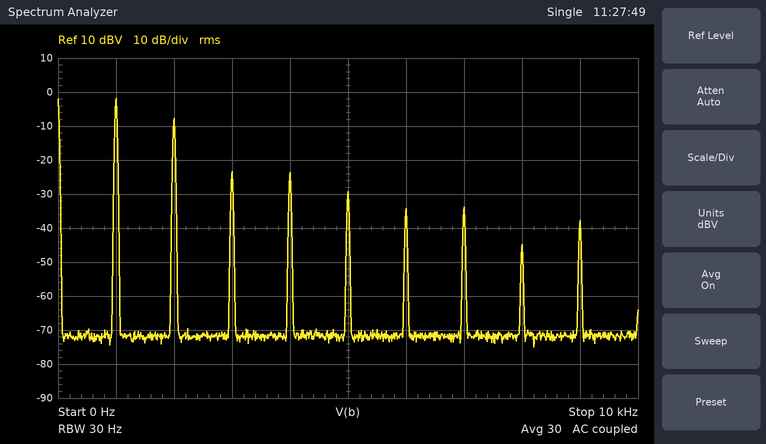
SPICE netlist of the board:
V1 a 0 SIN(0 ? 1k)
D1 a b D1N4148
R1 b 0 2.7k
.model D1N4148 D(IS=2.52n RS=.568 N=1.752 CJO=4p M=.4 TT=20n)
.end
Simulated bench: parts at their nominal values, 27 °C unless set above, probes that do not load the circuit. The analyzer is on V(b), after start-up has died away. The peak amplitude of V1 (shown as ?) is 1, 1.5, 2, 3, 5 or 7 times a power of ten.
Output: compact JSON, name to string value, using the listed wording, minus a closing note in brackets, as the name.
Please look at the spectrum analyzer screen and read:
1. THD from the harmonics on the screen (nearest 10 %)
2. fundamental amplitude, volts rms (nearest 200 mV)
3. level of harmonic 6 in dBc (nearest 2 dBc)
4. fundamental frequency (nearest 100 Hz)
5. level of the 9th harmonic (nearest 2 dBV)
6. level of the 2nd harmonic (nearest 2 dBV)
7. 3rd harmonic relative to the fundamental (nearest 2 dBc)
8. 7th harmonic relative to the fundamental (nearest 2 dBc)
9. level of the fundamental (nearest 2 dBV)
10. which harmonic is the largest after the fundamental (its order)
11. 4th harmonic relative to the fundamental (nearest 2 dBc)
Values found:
{"THD from the harmonics on the screen": "50 %", "fundamental amplitude, volts rms": "800 mV", "level of harmonic 6 in dBc": "-32 dBc", "fundamental frequency": "1.0 kHz", "level of the 9th harmonic": "-38 dBV", "level of the 2nd harmonic": "-8 dBV", "3rd harmonic relative to the fundamental": "-22 dBc", "7th harmonic relative to the fundamental": "-32 dBc", "level of the fundamental": "-2 dBV", "which harmonic is the largest after the fundamental": "2", "4th harmonic relative to the fundamental": "-22 dBc"}
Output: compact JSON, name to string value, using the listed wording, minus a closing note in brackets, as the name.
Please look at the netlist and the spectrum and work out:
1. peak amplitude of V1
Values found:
{"peak amplitude of V1": "3 V"}
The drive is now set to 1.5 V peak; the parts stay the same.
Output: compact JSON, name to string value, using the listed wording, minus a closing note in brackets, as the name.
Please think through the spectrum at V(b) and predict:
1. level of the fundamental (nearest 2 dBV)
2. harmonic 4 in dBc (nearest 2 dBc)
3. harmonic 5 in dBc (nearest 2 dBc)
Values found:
{"level of the fundamental": "-10 dBV", "harmonic 4 in dBc": "-26 dBc", "harmonic 5 in dBc": "-24 dBc"}
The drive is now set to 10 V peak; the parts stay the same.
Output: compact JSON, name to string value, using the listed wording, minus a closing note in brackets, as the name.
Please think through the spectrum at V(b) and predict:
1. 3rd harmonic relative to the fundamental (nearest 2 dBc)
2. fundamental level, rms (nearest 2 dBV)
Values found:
{"3rd harmonic relative to the fundamental": "-32 dBc", "fundamental level, rms": "10 dBV"}
